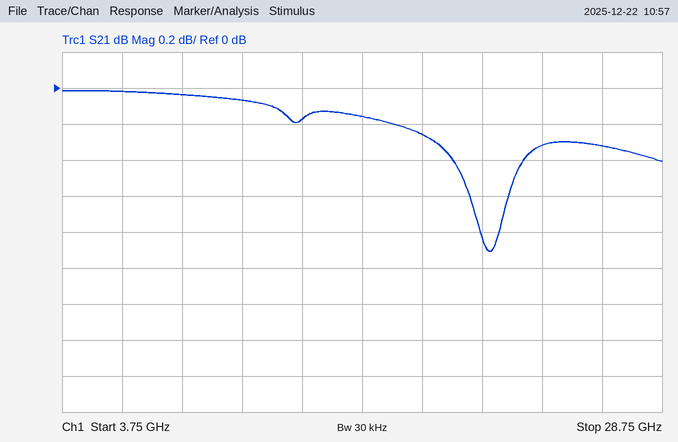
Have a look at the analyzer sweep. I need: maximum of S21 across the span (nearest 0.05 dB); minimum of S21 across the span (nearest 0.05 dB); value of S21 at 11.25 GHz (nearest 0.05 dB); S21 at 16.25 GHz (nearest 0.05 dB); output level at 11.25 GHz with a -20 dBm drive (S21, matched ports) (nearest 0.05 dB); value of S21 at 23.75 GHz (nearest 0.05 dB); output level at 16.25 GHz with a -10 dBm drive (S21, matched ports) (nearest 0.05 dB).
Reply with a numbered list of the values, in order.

1. 0.00 dB
2. -0.90 dB
3. -0.05 dB
4. -0.15 dB
5. -20.05 dBm
6. -0.30 dB
7. -10.15 dBm
